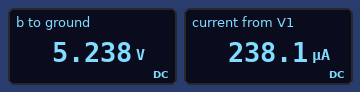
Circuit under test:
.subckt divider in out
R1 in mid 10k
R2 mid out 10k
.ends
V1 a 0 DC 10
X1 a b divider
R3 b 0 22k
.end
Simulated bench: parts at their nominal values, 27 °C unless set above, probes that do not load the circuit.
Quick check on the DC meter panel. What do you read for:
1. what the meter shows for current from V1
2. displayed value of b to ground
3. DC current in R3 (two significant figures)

238.1 µA
5.238 V
240 µA
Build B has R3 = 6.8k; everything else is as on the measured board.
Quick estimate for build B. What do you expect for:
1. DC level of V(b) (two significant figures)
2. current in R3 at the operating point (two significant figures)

2.5 V
370 µA
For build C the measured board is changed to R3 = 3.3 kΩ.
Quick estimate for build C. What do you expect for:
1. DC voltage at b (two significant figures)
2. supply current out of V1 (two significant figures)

1.4 V
430 µA
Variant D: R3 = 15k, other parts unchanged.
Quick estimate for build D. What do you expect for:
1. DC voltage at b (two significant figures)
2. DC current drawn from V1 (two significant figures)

4.3 V
290 µA
